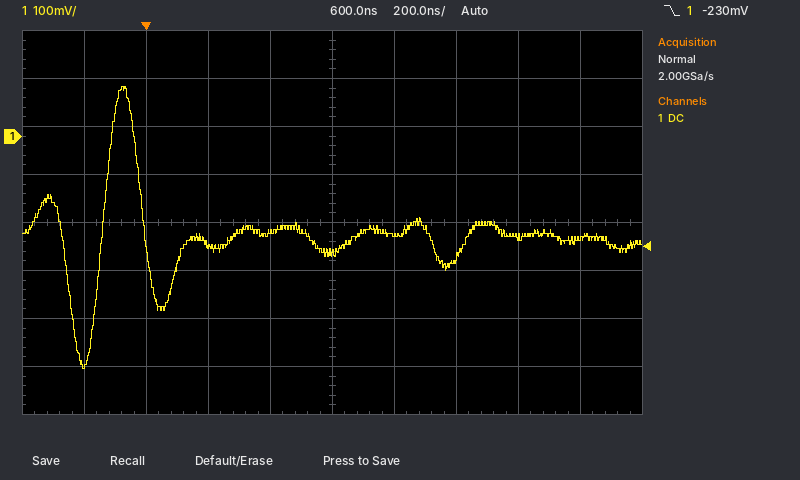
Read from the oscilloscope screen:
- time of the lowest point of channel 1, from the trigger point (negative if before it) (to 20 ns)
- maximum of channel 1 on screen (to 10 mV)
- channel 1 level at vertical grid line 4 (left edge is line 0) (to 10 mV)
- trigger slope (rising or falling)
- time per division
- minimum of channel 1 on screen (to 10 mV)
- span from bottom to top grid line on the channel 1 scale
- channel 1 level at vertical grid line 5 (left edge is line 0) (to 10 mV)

-200 ns
100 mV
-200 mV
falling
200 ns
-480 mV
800 mV
-240 mV
